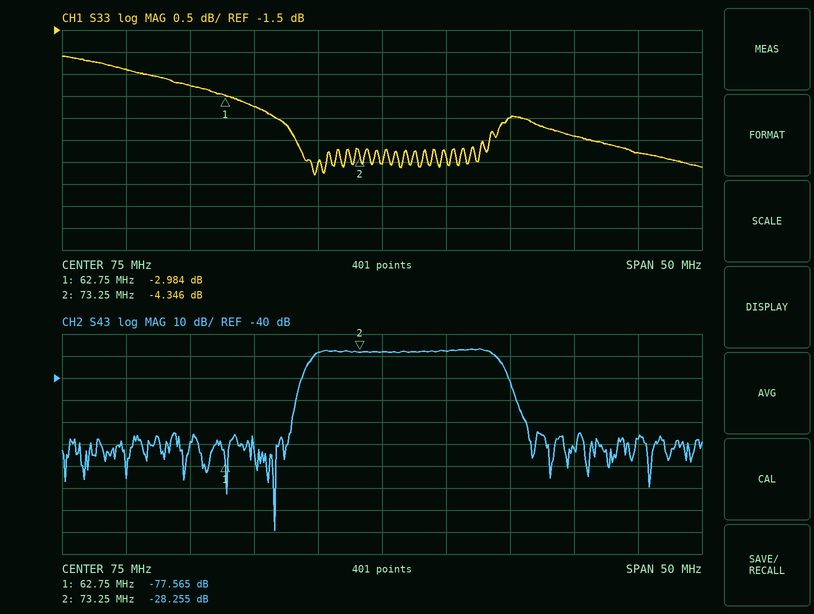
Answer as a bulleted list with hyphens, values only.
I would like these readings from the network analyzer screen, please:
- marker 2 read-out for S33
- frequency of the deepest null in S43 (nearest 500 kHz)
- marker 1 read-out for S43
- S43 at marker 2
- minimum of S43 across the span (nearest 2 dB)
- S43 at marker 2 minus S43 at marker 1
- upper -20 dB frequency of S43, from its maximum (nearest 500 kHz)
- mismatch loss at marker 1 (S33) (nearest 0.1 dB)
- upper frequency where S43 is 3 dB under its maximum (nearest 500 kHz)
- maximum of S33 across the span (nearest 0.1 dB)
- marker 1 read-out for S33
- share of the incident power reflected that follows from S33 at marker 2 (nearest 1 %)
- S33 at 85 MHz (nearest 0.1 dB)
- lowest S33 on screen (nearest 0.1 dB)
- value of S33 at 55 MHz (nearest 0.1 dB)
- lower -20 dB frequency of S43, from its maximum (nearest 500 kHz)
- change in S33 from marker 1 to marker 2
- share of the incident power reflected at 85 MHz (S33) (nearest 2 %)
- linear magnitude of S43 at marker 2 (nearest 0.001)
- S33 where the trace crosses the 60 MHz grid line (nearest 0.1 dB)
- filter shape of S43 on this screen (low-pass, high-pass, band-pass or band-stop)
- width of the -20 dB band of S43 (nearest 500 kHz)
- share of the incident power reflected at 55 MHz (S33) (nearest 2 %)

- -4.346 dB
- 66.5 MHz
- -77.565 dB
- -28.255 dB
- -110 dB
- 49.310 dB
- 85.5 MHz
- 3.0 dB
- 84.0 MHz
- -2.1 dB
- -2.984 dB
- 37 %
- -3.5 dB
- -4.8 dB
- -2.4 dB
- 68.5 MHz
- -1.362 dB
- 44 %
- 0.039
- -2.8 dB
- band-pass
- 17.0 MHz
- 58 %
